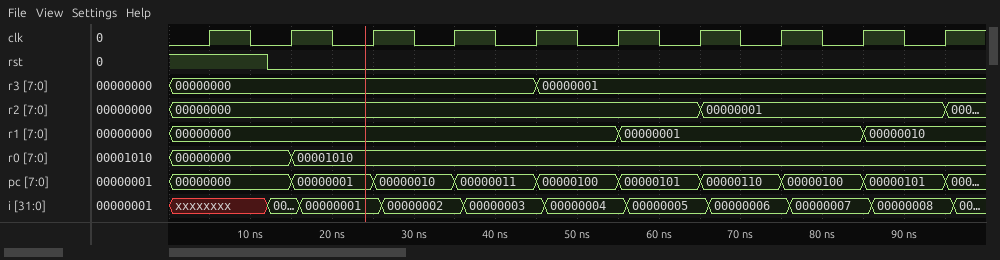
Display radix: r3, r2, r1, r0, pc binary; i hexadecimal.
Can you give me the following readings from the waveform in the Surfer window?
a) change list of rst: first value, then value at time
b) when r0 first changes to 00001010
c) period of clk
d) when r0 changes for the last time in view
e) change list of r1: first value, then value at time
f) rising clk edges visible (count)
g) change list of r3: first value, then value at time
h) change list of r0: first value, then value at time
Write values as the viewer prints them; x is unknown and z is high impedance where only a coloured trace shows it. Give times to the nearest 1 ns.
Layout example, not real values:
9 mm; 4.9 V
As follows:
1, 0 at 12 ns; 15 ns; 10 ns; 15 ns; 00000000, 00000001 at 55 ns, 00000010 at 85 ns; 10; 00000000, 00000001 at 45 ns; 00000000, 00001010 at 15 ns
